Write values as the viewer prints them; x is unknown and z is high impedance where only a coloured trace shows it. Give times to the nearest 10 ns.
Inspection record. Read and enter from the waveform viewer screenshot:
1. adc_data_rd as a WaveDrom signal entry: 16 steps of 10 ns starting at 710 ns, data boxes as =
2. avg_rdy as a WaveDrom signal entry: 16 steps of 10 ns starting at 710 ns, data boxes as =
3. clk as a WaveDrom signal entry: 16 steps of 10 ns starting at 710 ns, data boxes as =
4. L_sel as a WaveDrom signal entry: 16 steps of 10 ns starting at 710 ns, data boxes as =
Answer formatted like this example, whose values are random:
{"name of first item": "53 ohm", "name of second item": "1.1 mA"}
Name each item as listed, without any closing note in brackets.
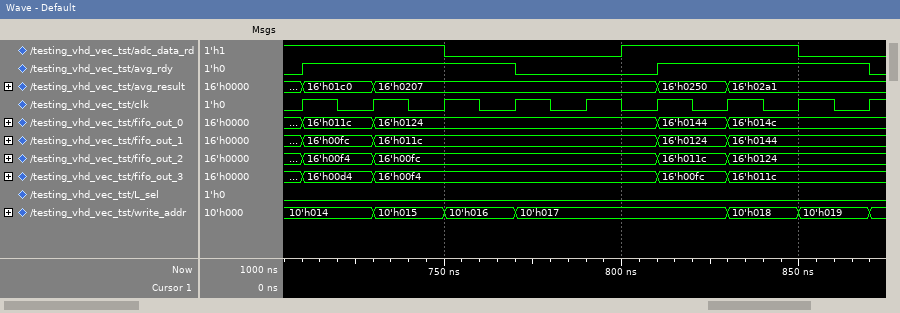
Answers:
{"adc_data_rd as a WaveDrom signal entry: 16 steps of 10 ns starting at 710 ns, data boxes as =": "{name: 'adc_data_rd', wave: '1...0....1....0.'}", "avg_rdy as a WaveDrom signal entry: 16 steps of 10 ns starting at 710 ns, data boxes as =": "{name: 'avg_rdy', wave: '1.....0...1.....'}", "clk as a WaveDrom signal entry: 16 steps of 10 ns starting at 710 ns, data boxes as =": "{name: 'clk', wave: '1010101010101010'}", "L_sel as a WaveDrom signal entry: 16 steps of 10 ns starting at 710 ns, data boxes as =": "{name: 'L_sel', wave: '0...............'}"}
